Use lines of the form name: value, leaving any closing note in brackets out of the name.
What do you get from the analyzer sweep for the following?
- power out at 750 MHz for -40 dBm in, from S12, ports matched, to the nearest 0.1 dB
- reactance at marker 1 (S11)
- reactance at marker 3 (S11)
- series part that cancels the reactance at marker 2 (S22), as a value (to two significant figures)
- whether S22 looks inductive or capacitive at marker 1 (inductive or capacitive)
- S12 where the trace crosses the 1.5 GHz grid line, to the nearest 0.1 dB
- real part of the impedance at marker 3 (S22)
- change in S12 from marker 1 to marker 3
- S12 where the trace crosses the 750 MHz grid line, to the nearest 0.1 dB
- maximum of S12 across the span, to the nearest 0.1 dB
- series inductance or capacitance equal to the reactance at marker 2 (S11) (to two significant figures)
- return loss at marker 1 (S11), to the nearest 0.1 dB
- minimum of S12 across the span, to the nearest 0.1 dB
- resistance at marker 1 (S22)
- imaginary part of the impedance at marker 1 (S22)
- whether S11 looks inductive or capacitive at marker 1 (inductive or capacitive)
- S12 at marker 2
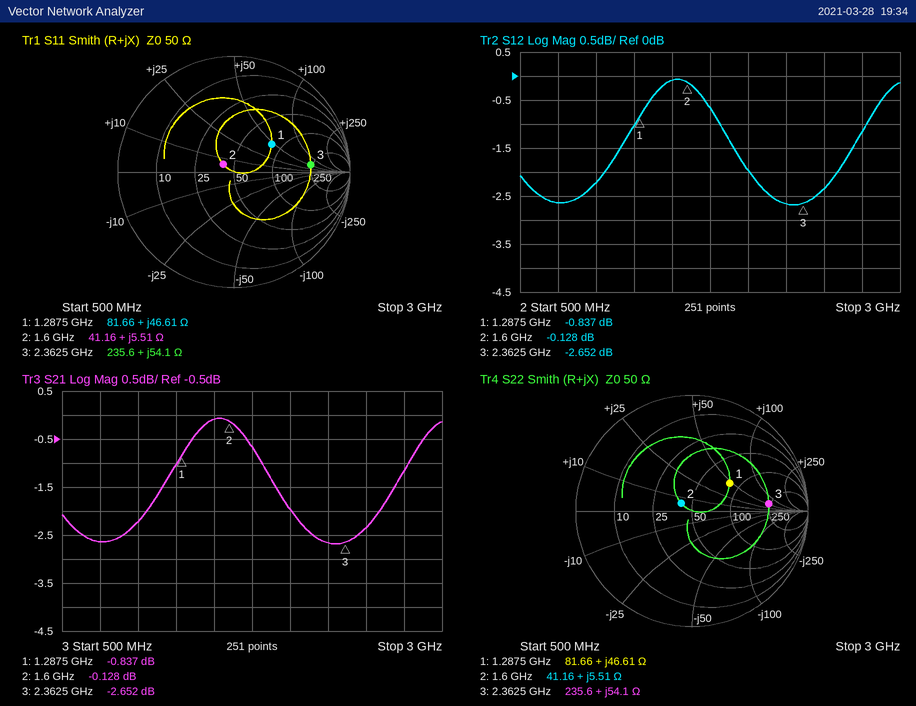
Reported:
power out at 750 MHz for -40 dBm in, from S12, ports matched, to the nearest 0.1 dB: -42.6 dBm
reactance at marker 1: +46.61 Ω
reactance at marker 3: +54.1 Ω
series part that cancels the reactance at marker 2 (S22), as a value: 18 pF
whether S22 looks inductive or capacitive at marker 1: inductive
S12 where the trace crosses the 1.5 GHz grid line, to the nearest 0.1 dB: -0.1 dB
real part of the impedance at marker 3: 235.6 Ω
change in S12 from marker 1 to marker 3: -1.815 dB
S12 where the trace crosses the 750 MHz grid line, to the nearest 0.1 dB: -2.6 dB
maximum of S12 across the span, to the nearest 0.1 dB: -0.1 dB
series inductance or capacitance equal to the reactance at marker 2 (S11): 550 pH
return loss at marker 1 (S11), to the nearest 0.1 dB: 7.9 dB
minimum of S12 across the span, to the nearest 0.1 dB: -2.7 dB
resistance at marker 1: 81.66 Ω
imaginary part of the impedance at marker 1: +46.61 Ω
whether S11 looks inductive or capacitive at marker 1: inductive
S12 at marker 2: -0.128 dB
